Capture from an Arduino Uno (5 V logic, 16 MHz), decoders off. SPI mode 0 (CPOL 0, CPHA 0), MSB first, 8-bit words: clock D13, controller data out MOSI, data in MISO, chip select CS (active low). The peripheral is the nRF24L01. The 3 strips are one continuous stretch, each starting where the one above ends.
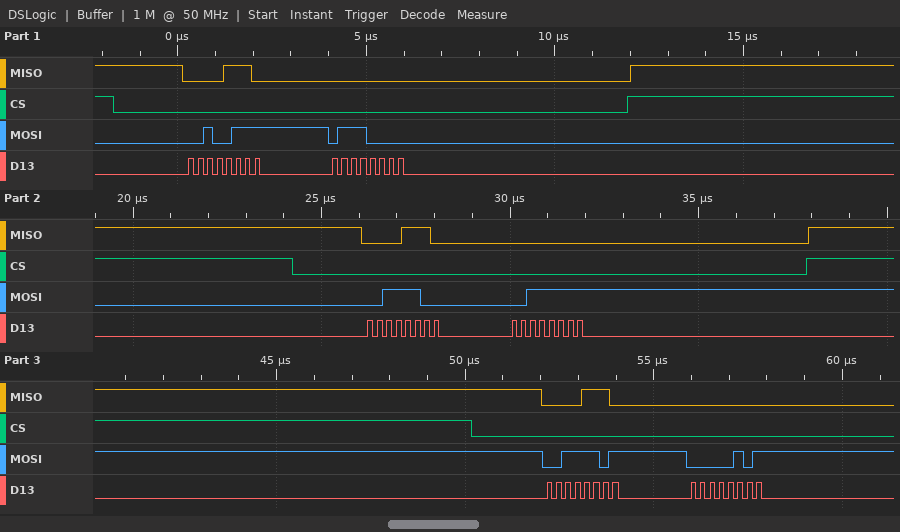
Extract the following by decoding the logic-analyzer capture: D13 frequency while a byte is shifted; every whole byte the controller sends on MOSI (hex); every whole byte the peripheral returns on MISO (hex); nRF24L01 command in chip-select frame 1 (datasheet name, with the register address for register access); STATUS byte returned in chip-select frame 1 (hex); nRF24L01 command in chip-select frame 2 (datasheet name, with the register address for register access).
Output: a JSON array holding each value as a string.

["4 MHz", "27 70 3C 3F 3D 05", "0E 00 0E 00 0E 00", "W_REGISTER 0x07", "0x0E", "W_REGISTER 0x1C"]
